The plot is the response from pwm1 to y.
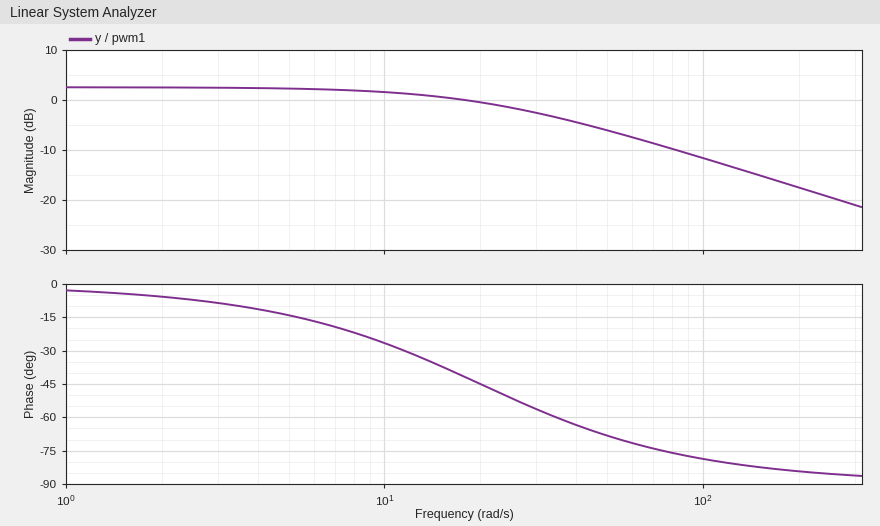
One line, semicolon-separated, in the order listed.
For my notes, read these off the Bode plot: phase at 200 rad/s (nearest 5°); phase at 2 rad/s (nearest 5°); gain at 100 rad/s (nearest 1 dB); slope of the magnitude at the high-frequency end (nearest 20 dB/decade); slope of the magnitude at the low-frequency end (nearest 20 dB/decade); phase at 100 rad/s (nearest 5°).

-85°; -5°; -12 dB; -20 dB/decade; 0 dB/decade; -80°
